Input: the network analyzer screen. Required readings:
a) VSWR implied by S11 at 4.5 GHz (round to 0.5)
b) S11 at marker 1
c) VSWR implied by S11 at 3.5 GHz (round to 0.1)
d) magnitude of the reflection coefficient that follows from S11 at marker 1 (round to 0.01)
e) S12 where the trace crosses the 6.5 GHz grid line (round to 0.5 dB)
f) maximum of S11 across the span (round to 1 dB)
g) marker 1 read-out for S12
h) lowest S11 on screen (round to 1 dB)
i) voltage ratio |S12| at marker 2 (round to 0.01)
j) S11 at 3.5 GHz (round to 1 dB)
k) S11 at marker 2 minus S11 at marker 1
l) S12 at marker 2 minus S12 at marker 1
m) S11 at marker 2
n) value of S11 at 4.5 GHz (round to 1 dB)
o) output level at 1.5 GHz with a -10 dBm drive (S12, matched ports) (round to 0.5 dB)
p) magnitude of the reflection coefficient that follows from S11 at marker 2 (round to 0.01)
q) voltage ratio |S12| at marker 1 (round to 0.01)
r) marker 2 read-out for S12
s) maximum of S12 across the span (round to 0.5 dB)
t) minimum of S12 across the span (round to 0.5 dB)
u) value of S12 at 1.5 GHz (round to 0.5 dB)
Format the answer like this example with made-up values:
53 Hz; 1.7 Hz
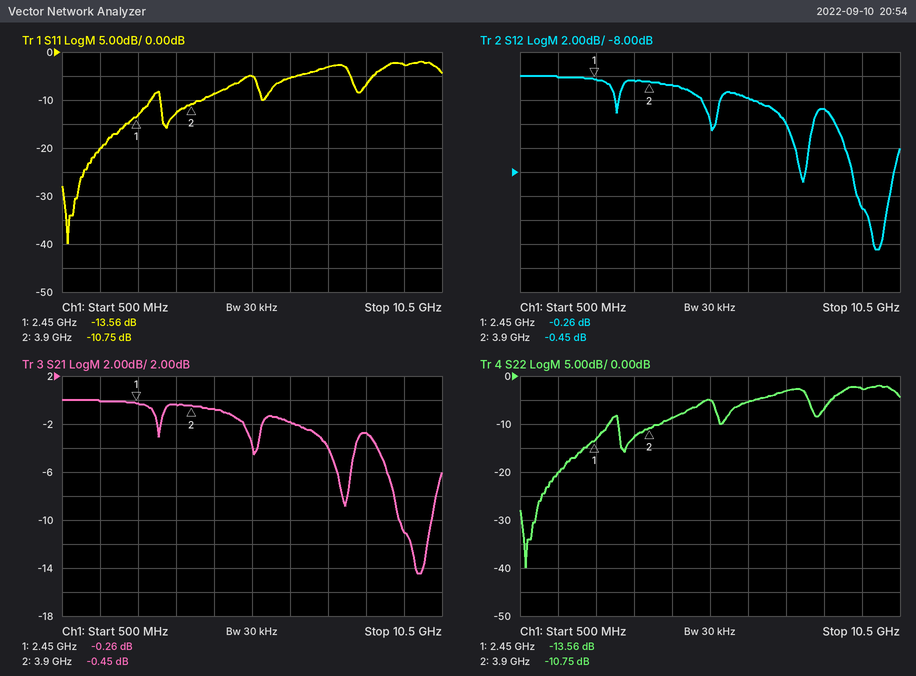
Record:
2.0; -13.56 dB; 1.6; 0.21; -2.0 dB; -2 dB; -0.26 dB; -40 dB; 0.95; -13 dB; 2.81 dB; -0.19 dB; -10.75 dB; -9 dB; -10.0 dBm; 0.29; 0.97; -0.45 dB; 0.0 dB; -14.5 dB; 0.0 dB
